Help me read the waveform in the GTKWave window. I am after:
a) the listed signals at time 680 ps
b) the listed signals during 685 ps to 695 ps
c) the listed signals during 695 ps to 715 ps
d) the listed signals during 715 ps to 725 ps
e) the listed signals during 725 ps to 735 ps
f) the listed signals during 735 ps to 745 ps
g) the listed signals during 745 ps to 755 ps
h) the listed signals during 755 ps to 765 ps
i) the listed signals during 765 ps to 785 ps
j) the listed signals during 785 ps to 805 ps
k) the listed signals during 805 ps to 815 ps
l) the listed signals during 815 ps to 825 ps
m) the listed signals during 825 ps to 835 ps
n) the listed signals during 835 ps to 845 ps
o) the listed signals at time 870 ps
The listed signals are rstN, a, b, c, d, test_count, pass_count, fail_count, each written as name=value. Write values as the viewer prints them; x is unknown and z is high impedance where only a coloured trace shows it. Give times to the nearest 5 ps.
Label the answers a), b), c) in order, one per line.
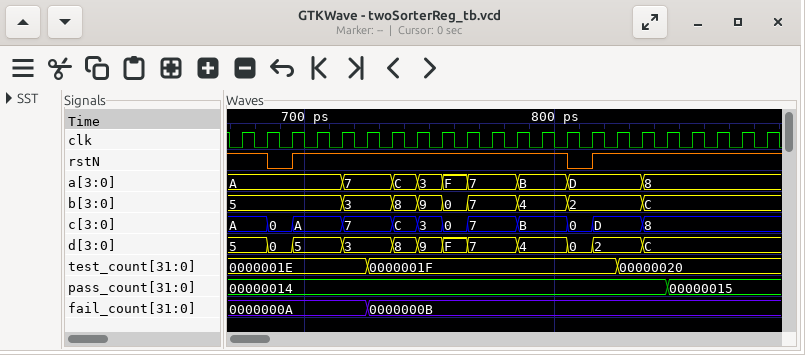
a) rstN=1, a=A, b=5, c=A, d=5, test_count=0000001E, pass_count=00000014, fail_count=0000000A
b) rstN=0, a=A, b=5, c=0, d=0, test_count=0000001E, pass_count=00000014, fail_count=0000000A
c) rstN=1, a=A, b=5, c=A, d=5, test_count=0000001E, pass_count=00000014, fail_count=0000000A
d) rstN=1, a=7, b=3, c=7, d=3, test_count=0000001E, pass_count=00000014, fail_count=0000000A
e) rstN=1, a=7, b=3, c=7, d=3, test_count=0000001F, pass_count=00000014, fail_count=0000000B
f) rstN=1, a=C, b=8, c=C, d=8, test_count=0000001F, pass_count=00000014, fail_count=0000000B
g) rstN=1, a=3, b=9, c=3, d=9, test_count=0000001F, pass_count=00000014, fail_count=0000000B
h) rstN=1, a=F, b=0, c=0, d=F, test_count=0000001F, pass_count=00000014, fail_count=0000000B
i) rstN=1, a=7, b=7, c=7, d=7, test_count=0000001F, pass_count=00000014, fail_count=0000000B
j) rstN=1, a=B, b=4, c=B, d=4, test_count=0000001F, pass_count=00000014, fail_count=0000000B
k) rstN=0, a=D, b=2, c=0, d=0, test_count=0000001F, pass_count=00000014, fail_count=0000000B
l) rstN=1, a=D, b=2, c=D, d=2, test_count=0000001F, pass_count=00000014, fail_count=0000000B
m) rstN=1, a=D, b=2, c=D, d=2, test_count=00000020, pass_count=00000014, fail_count=0000000B
n) rstN=1, a=8, b=C, c=8, d=C, test_count=00000020, pass_count=00000014, fail_count=0000000B
o) rstN=1, a=8, b=C, c=8, d=C, test_count=00000020, pass_count=00000015, fail_count=0000000B
